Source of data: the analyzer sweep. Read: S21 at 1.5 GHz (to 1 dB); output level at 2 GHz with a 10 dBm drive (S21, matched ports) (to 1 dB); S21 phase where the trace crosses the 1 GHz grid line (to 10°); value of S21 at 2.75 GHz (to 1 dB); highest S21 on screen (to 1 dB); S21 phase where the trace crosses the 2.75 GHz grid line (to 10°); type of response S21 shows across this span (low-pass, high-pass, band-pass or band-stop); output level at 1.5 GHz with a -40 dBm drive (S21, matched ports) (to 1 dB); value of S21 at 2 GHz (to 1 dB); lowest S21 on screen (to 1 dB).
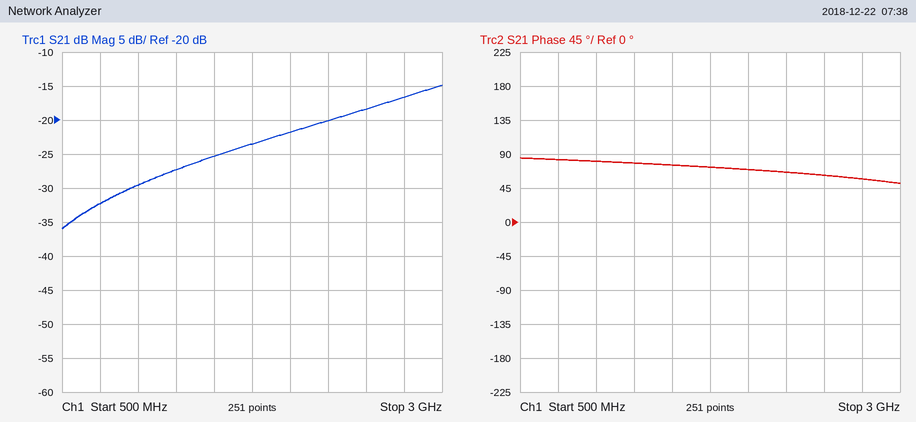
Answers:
-25 dB
-12 dBm
80°
-17 dB
-15 dB
60°
high-pass
-65 dBm
-22 dB
-36 dB
